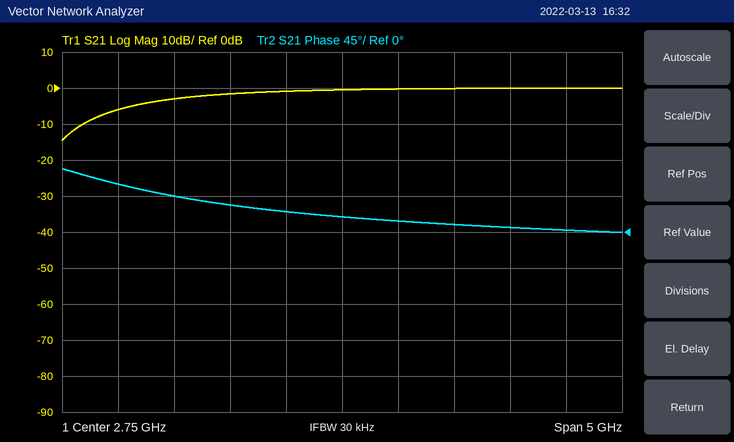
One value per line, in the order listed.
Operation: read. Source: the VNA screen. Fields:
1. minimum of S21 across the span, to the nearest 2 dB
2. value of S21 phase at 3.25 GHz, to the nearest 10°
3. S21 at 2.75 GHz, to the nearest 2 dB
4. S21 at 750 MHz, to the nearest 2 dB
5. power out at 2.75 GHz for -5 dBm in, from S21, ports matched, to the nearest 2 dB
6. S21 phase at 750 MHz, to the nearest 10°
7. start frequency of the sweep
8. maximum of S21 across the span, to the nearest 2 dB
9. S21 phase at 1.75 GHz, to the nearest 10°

-14 dB
10°
0 dB
-6 dB
-6 dBm
60°
250 MHz
0 dB
30°
